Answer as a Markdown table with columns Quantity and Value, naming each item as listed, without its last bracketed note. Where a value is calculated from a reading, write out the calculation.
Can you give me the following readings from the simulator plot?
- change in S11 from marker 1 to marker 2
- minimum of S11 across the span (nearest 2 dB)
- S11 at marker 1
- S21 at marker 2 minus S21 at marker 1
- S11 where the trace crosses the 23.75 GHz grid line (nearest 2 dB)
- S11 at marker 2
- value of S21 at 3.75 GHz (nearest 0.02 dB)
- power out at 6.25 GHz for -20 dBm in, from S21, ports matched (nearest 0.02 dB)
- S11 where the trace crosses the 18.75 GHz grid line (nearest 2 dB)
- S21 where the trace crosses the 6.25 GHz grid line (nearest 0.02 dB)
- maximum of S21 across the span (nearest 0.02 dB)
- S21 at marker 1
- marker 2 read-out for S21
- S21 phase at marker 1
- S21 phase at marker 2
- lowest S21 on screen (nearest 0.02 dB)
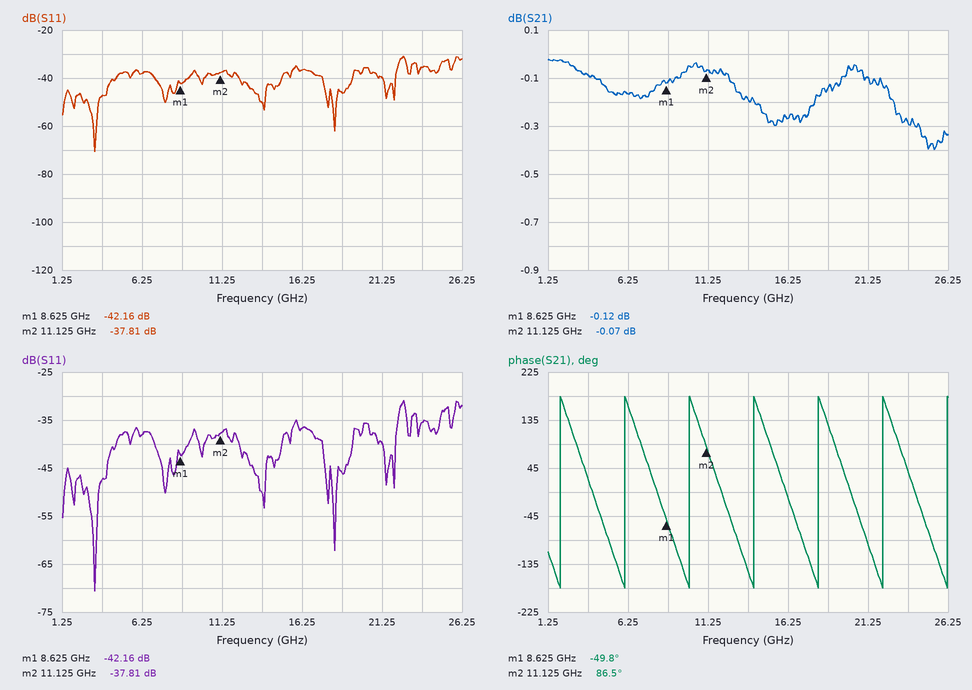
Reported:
| Quantity | Value |
|---|---|
| change in S11 from marker 1 to marker 2 | -37.81 − (-42.16) = 4.35 dB |
| minimum of S11 across the span | -70 dB |
| S11 at marker 1 | -42.16 dB |
| S21 at marker 2 minus S21 at marker 1 | -0.07 − (-0.12) = 0.05 dB |
| S11 where the trace crosses the 23.75 GHz grid line | -36 dB |
| S11 at marker 2 | -37.81 dB |
| value of S21 at 3.75 GHz | -0.08 dB |
| power out at 6.25 GHz for -20 dBm in, from S21, ports matched | -20 dBm + (-0.16 dB) = -20.16 dBm |
| S11 where the trace crosses the 18.75 GHz grid line | -46 dB |
| S21 where the trace crosses the 6.25 GHz grid line | -0.16 dB |
| maximum of S21 across the span | -0.02 dB |
| S21 at marker 1 | -0.12 dB |
| marker 2 read-out for S21 | -0.07 dB |
| S21 phase at marker 1 | -49.8° |
| S21 phase at marker 2 | 86.5° |
| lowest S21 on screen | -0.40 dB |
